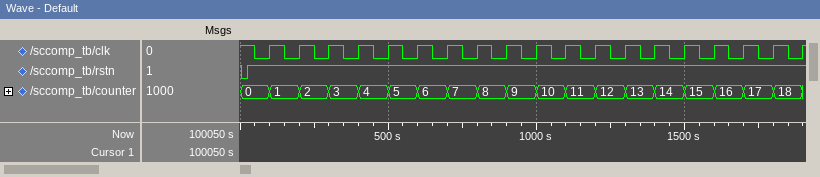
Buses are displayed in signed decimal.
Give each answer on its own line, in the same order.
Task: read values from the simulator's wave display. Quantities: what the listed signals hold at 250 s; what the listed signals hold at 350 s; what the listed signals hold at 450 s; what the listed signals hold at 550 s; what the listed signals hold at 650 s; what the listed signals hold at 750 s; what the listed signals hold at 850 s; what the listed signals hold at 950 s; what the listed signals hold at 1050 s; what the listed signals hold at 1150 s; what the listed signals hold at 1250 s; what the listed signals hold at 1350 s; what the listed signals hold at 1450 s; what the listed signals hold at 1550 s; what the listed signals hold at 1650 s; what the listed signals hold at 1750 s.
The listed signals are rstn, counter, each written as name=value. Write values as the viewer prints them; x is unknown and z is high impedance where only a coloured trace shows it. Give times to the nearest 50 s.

rstn=1, counter=2
rstn=1, counter=3
rstn=1, counter=4
rstn=1, counter=5
rstn=1, counter=6
rstn=1, counter=7
rstn=1, counter=8
rstn=1, counter=9
rstn=1, counter=10
rstn=1, counter=11
rstn=1, counter=12
rstn=1, counter=13
rstn=1, counter=14
rstn=1, counter=15
rstn=1, counter=16
rstn=1, counter=17
